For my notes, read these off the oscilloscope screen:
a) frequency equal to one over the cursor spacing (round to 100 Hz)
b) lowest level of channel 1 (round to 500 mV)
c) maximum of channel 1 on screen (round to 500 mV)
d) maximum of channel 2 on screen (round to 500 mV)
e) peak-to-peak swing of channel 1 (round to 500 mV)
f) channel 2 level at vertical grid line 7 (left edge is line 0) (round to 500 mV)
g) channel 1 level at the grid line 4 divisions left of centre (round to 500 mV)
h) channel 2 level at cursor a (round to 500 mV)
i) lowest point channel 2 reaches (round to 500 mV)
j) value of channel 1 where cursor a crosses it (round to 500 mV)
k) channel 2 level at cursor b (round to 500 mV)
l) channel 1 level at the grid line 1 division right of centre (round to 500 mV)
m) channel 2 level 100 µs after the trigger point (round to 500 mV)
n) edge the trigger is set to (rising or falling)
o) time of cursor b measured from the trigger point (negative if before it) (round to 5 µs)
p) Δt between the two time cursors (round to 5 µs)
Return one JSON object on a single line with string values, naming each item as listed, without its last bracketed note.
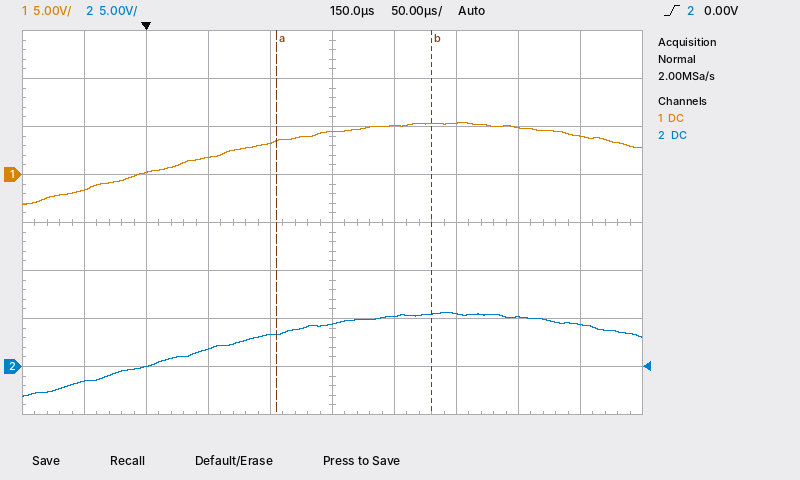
{"frequency equal to one over the cursor spacing": "8.0 kHz", "lowest level of channel 1": "-3.0 V", "maximum of channel 1 on screen": "5.5 V", "maximum of channel 2 on screen": "5.5 V", "peak-to-peak swing of channel 1": "8.5 V", "channel 2 level at vertical grid line 7 (left edge is line 0)": "5.5 V", "channel 1 level at the grid line 4 divisions left of centre": "-1.5 V", "channel 2 level at cursor a": "3.5 V", "lowest point channel 2 reaches": "-3.0 V", "value of channel 1 where cursor a crosses it": "3.5 V", "channel 2 level at cursor b": "5.5 V", "channel 1 level at the grid line 1 division right of centre": "5.0 V", "channel 2 level 100 µs after the trigger point": "3.5 V", "edge the trigger is set to": "rising", "time of cursor b measured from the trigger point (negative if before it)": "+230 µs", "Δt between the two time cursors": "125 µs"}
